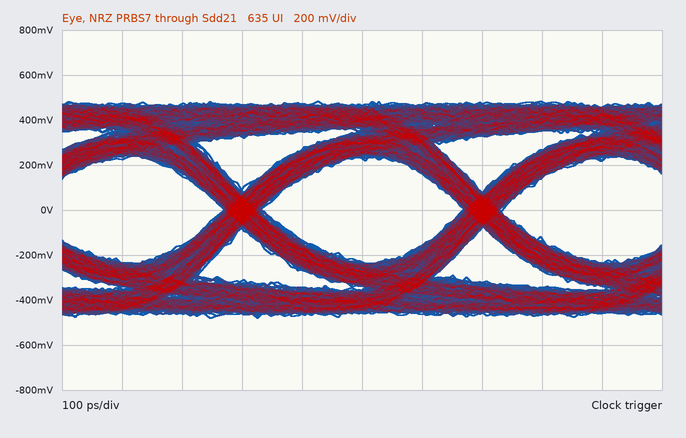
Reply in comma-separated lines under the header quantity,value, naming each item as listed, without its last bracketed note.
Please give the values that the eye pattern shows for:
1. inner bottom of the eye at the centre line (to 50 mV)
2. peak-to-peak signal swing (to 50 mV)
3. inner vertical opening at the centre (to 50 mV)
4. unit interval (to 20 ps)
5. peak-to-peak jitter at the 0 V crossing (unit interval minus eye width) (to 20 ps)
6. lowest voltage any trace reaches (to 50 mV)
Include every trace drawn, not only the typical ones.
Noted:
quantity,value
inner bottom of the eye at the centre line,-250 mV
peak-to-peak signal swing,950 mV
inner vertical opening at the centre,450 mV
unit interval,400 ps
peak-to-peak jitter at the 0 V crossing (unit interval minus eye width),60 ps
lowest voltage any trace reaches,-500 mV
